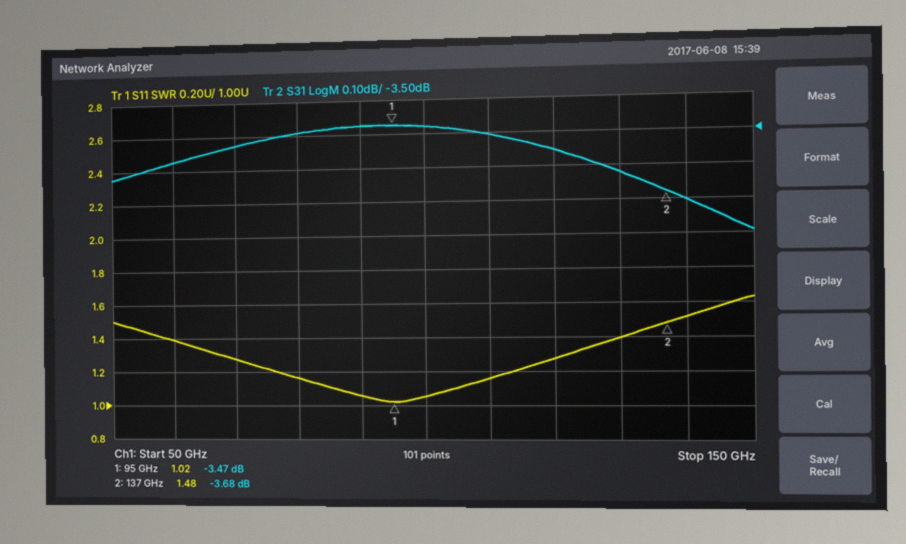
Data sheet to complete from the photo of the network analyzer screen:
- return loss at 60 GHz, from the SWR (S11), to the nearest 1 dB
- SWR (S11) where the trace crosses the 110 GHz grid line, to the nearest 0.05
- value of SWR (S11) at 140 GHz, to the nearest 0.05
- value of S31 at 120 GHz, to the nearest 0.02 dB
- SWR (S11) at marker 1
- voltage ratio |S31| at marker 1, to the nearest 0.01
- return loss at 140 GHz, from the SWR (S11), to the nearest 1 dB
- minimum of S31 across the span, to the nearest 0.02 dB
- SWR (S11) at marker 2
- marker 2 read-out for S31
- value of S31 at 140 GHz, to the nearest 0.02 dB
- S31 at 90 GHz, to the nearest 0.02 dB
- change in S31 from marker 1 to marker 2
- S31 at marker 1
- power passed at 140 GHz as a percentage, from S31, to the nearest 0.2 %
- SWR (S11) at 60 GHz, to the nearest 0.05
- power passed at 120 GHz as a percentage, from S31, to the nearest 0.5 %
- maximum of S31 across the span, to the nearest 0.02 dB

16 dB
1.15
1.50
-3.56 dB
1.02
0.67
14 dB
-3.80 dB
1.48
-3.68 dB
-3.70 dB
-3.48 dB
-0.21 dB
-3.47 dB
42.6 %
1.40
44.0 %
-3.48 dB
